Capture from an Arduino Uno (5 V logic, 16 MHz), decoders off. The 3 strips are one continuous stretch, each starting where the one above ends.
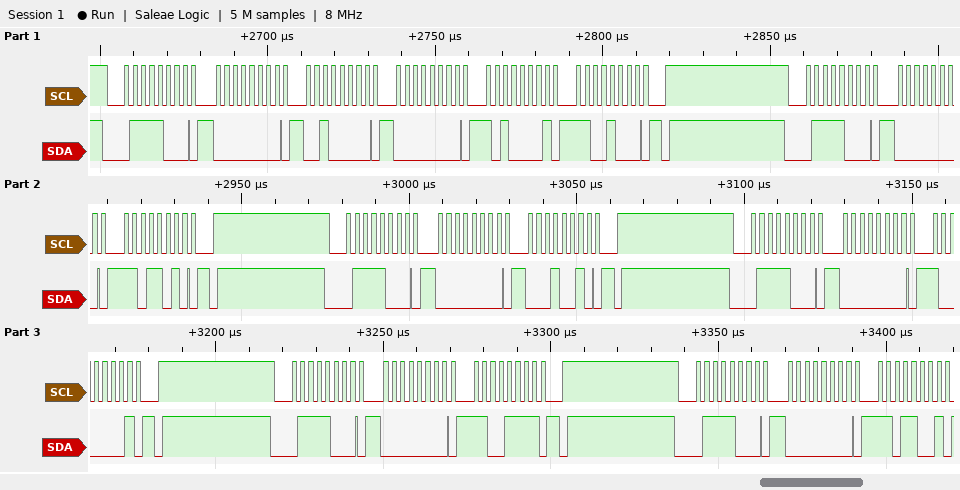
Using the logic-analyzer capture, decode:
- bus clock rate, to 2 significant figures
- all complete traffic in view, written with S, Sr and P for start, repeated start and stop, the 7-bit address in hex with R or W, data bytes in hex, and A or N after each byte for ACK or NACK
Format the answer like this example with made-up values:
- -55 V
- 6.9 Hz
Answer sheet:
- 400 kHz
- S 3CW A 00 A 20 A 00 A A1 A C8 A P S 3CW A 00 A DA A P S 3CW A 00 A 12 A P S 3CW A 00 A 81 A P S 3CW A 00 A CF A P S 3CW A 00 A D9 A
